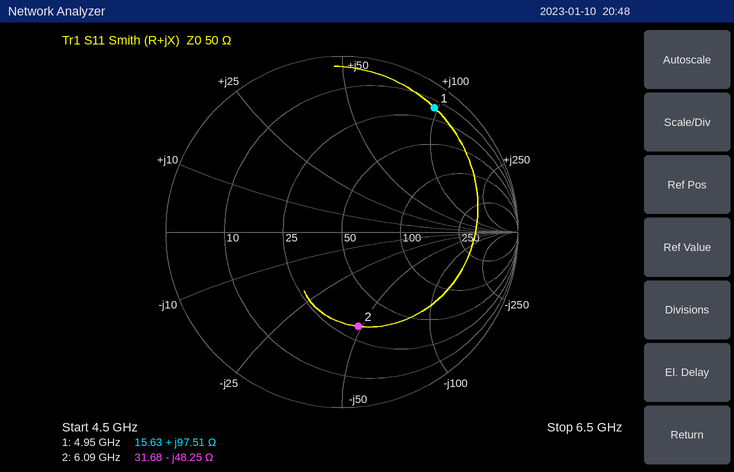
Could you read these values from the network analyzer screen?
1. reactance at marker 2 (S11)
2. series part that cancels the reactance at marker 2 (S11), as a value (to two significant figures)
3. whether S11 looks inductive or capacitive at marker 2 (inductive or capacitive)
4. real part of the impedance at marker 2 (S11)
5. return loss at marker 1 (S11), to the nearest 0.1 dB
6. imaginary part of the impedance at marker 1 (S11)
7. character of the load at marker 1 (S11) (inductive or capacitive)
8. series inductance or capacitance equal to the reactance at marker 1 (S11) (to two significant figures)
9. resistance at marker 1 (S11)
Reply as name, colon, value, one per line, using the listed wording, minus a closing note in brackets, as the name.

reactance at marker 2: -48.25 Ω
series part that cancels the reactance at marker 2 (S11), as a value: 1.3 nH
whether S11 looks inductive or capacitive at marker 2: capacitive
real part of the impedance at marker 2: 31.68 Ω
return loss at marker 1 (S11), to the nearest 0.1 dB: 1.1 dB
imaginary part of the impedance at marker 1: +97.51 Ω
character of the load at marker 1 (S11): inductive
series inductance or capacitance equal to the reactance at marker 1 (S11): 3.1 nH
resistance at marker 1: 15.63 Ω
